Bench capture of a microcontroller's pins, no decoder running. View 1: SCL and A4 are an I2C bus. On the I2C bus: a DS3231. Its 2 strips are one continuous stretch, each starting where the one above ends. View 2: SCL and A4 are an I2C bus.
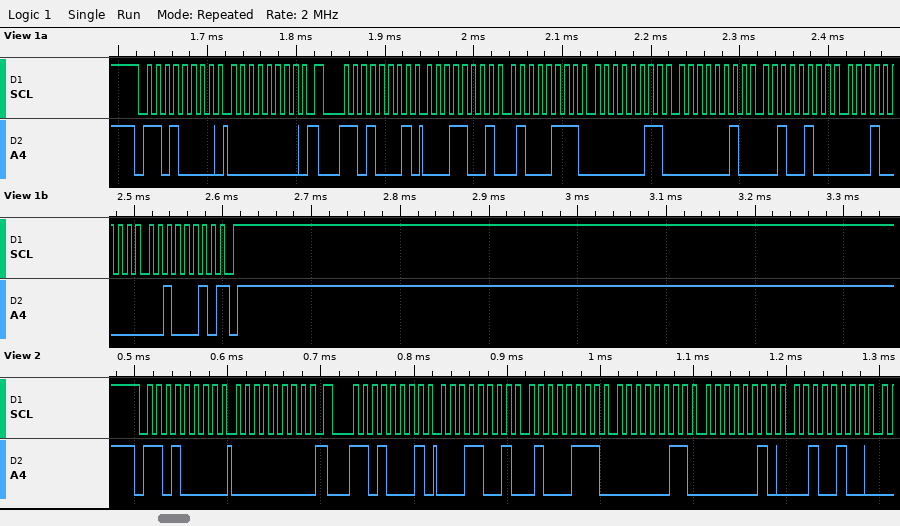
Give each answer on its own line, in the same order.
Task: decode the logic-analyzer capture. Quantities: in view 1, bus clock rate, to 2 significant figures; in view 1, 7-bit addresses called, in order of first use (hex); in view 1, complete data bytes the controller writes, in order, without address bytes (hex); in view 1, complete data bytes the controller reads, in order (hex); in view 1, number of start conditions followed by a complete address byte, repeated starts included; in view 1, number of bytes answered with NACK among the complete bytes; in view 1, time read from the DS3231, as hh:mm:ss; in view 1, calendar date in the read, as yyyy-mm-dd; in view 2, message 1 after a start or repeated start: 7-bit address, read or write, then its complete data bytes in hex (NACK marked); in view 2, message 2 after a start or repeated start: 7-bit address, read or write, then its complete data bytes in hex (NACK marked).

100 kHz
0x68
00
19 47 03 02 24 10 22
2
1
03:47:19
2022-10-24
0x68 write: 00
0x68 read: 19 47 03 02 24
